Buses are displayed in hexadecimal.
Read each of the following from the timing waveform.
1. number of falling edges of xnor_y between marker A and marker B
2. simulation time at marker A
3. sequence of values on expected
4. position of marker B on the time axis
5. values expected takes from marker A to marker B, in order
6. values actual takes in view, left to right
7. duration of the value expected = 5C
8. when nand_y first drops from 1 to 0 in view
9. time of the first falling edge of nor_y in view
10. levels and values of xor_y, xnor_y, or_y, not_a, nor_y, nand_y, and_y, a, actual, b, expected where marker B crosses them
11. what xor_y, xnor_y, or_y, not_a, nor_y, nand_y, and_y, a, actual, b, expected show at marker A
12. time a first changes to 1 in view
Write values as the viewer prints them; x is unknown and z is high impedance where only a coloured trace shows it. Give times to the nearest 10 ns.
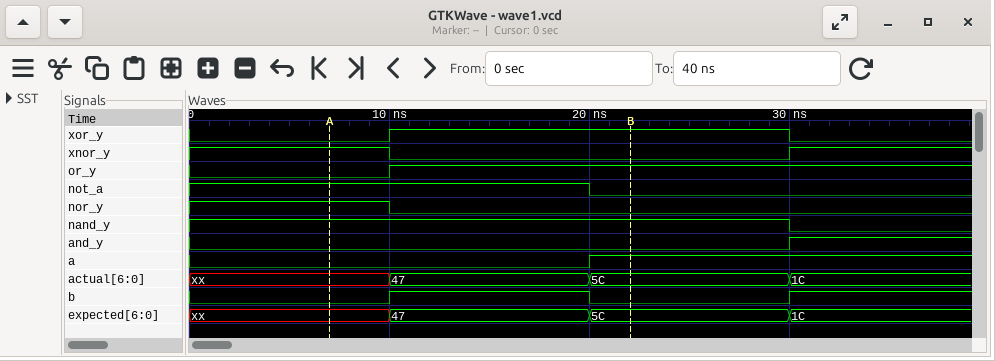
1
10 ns
xx, 47, 5C, 1C
20 ns
xx, 47, 5C
xx, 47, 5C, 1C
10 ns
30 ns
10 ns
xor_y=1, xnor_y=0, or_y=1, not_a=0, nor_y=0, nand_y=1, and_y=0, a=1, actual=5C, b=0, expected=5C
xor_y=0, xnor_y=1, or_y=0, not_a=1, nor_y=1, nand_y=1, and_y=0, a=0, actual=xx, b=0, expected=xx
20 ns
